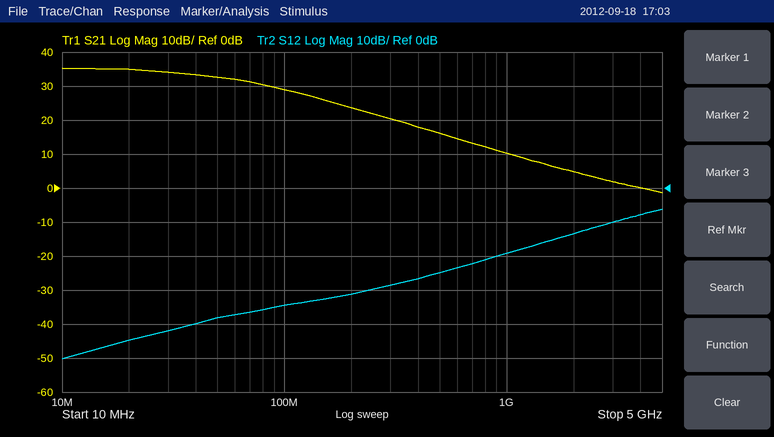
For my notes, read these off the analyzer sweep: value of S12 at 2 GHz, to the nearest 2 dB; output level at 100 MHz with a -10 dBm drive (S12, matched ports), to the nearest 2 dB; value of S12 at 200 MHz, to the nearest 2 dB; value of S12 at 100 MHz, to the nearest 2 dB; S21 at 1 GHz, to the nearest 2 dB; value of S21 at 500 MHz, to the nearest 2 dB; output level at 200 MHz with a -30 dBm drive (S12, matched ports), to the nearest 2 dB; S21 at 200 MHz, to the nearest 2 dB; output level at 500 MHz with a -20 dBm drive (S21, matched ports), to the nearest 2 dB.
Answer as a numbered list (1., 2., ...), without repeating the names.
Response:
1. -14 dB
2. -44 dBm
3. -32 dB
4. -34 dB
5. 10 dB
6. 16 dB
7. -62 dBm
8. 24 dB
9. -4 dBm
